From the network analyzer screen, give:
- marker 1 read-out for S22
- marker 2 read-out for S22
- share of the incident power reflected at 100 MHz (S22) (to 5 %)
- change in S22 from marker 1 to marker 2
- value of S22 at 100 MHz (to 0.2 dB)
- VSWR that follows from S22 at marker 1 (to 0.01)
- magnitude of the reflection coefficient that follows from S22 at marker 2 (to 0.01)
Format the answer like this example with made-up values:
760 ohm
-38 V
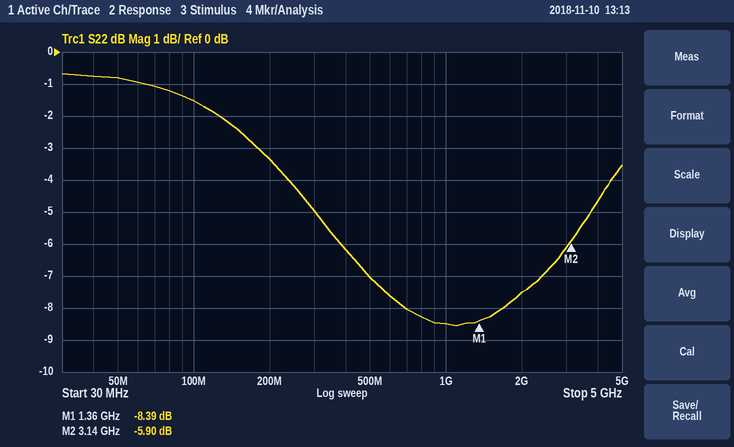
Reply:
-8.39 dB
-5.90 dB
70 %
2.49 dB
-1.6 dB
2.23
0.51
